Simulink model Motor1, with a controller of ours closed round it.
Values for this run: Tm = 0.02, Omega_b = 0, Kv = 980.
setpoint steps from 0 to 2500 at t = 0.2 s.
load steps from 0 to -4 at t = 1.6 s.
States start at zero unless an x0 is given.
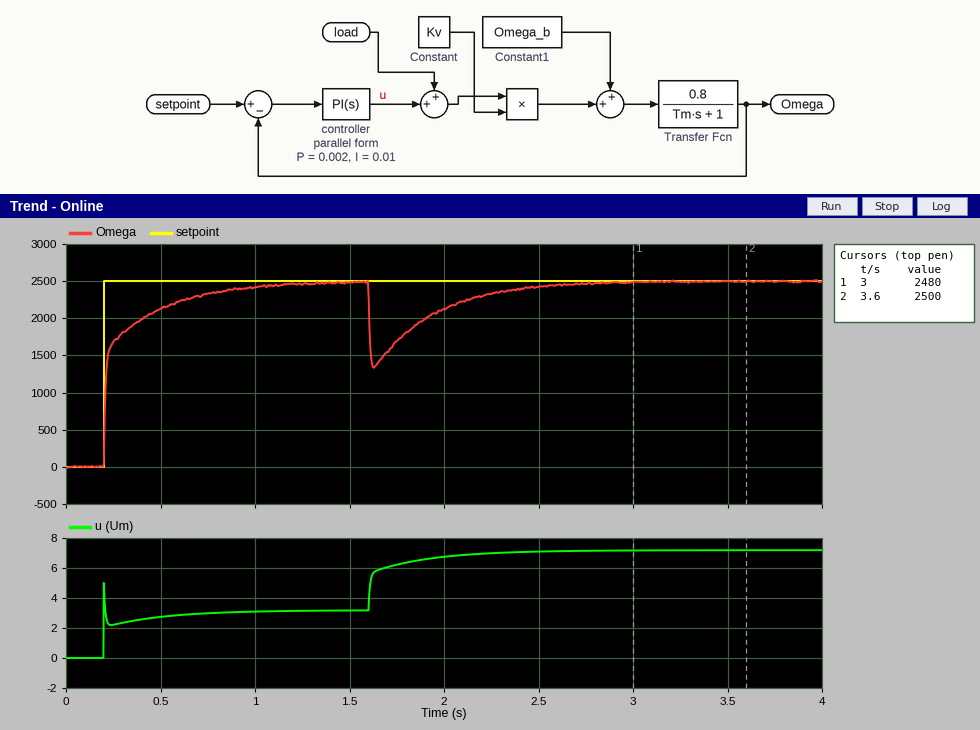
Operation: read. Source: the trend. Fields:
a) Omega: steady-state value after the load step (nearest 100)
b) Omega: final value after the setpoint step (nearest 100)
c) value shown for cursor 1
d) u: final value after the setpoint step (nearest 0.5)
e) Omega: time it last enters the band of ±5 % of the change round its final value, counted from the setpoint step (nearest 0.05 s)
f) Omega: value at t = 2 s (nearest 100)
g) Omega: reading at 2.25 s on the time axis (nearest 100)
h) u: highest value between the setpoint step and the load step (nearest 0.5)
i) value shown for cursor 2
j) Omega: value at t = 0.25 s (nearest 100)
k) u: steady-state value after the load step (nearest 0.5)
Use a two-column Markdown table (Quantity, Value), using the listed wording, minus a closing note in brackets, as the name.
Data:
| Quantity | Value |
|---|---|
| Omega: steady-state value after the load step | 2500 |
| Omega: final value after the setpoint step | 2500 |
| value shown for cursor 1 | 2480 |
| u: final value after the setpoint step | 3.0 |
| Omega: time it last enters the band of ±5 % of the change round its final value, counted from the setpoint step | 0.65 s |
| Omega: value at t = 2 s | 2100 |
| Omega: reading at 2.25 s on the time axis | 2300 |
| u: highest value between the setpoint step and the load step | 5.0 |
| value shown for cursor 2 | 2500 |
| Omega: value at t = 0.25 s | 1700 |
| u: steady-state value after the load step | 7.0 |
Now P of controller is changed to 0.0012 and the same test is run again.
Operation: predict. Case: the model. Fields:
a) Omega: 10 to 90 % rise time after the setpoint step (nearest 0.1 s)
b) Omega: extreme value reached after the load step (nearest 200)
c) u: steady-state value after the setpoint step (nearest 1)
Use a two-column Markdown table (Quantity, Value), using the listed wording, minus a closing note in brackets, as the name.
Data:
| Quantity | Value |
|---|---|
| Omega: 10 to 90 % rise time after the setpoint step | 0.4 s |
| Omega: extreme value reached after the load step | 1000 |
| u: steady-state value after the setpoint step | 3 |
